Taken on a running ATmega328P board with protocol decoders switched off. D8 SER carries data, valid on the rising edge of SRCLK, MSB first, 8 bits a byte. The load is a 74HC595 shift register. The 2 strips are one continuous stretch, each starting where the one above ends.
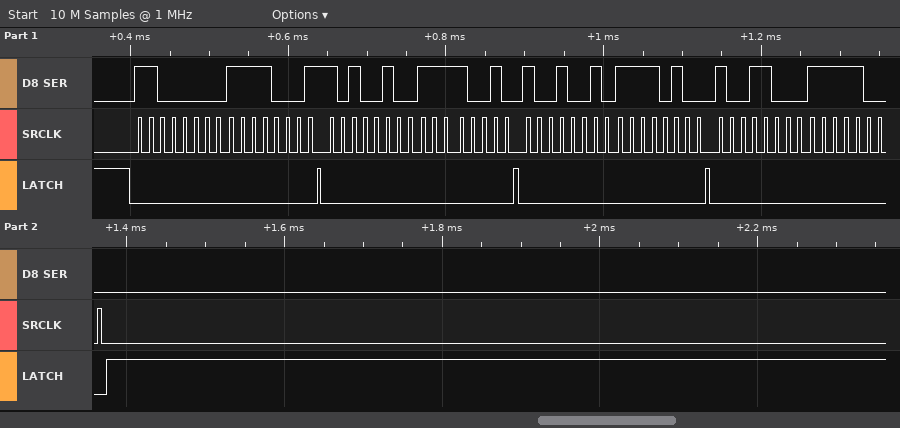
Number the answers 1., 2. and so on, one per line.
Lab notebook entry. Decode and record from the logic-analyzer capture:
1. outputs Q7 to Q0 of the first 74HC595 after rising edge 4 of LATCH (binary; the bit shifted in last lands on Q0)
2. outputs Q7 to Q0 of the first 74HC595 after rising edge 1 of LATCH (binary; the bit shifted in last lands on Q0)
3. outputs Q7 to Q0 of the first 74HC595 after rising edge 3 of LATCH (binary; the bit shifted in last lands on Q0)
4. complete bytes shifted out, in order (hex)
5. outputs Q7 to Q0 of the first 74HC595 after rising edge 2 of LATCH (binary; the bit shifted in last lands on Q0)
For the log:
1. 11111000
2. 11110001
3. 11110100
4. C0 F1 A4 F2 92 F4 98 F8
5. 11110010
